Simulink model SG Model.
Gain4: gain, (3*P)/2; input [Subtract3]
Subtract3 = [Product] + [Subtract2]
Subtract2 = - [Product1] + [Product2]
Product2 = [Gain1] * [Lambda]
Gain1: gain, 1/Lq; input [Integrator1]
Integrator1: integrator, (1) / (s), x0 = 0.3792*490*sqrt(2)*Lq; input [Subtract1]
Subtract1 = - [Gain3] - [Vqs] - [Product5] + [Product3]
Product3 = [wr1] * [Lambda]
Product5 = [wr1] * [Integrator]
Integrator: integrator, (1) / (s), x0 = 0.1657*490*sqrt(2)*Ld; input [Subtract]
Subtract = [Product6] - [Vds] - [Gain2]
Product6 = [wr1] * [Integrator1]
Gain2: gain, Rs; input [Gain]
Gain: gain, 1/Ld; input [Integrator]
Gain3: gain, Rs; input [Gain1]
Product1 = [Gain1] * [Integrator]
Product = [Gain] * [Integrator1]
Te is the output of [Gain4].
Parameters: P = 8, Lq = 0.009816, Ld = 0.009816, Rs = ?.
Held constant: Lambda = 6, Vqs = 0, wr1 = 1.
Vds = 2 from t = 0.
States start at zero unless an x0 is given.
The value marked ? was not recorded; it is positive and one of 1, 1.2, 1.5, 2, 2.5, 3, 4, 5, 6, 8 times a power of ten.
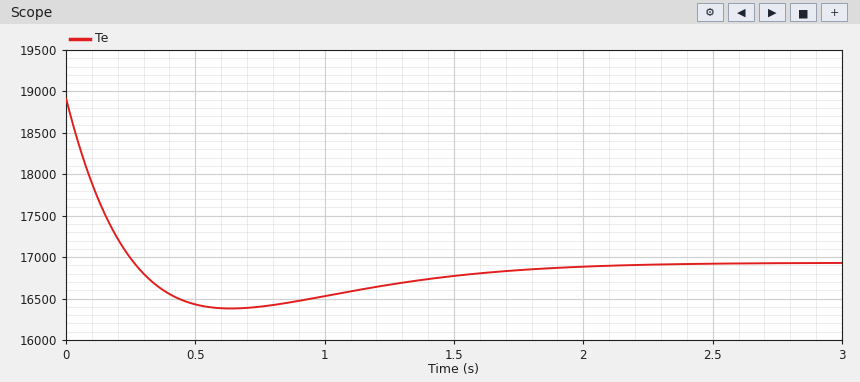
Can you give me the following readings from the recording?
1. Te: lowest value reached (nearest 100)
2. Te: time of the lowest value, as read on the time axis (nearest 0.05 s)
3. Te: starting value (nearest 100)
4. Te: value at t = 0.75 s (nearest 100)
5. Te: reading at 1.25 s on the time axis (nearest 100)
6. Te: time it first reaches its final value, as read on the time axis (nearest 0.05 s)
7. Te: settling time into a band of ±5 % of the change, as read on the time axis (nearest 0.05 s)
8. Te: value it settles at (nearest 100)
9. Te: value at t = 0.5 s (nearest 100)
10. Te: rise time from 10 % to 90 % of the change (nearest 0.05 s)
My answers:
16400
0.65 s
18900
16400
16700
0.25 s
1.70 s
16900
16400
0.20 s
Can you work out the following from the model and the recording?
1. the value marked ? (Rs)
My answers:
0.025
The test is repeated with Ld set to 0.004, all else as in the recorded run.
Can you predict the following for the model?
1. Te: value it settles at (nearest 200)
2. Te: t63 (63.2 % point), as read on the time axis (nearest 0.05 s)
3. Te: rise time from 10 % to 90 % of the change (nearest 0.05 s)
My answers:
17400
0.20 s
0.50 s
